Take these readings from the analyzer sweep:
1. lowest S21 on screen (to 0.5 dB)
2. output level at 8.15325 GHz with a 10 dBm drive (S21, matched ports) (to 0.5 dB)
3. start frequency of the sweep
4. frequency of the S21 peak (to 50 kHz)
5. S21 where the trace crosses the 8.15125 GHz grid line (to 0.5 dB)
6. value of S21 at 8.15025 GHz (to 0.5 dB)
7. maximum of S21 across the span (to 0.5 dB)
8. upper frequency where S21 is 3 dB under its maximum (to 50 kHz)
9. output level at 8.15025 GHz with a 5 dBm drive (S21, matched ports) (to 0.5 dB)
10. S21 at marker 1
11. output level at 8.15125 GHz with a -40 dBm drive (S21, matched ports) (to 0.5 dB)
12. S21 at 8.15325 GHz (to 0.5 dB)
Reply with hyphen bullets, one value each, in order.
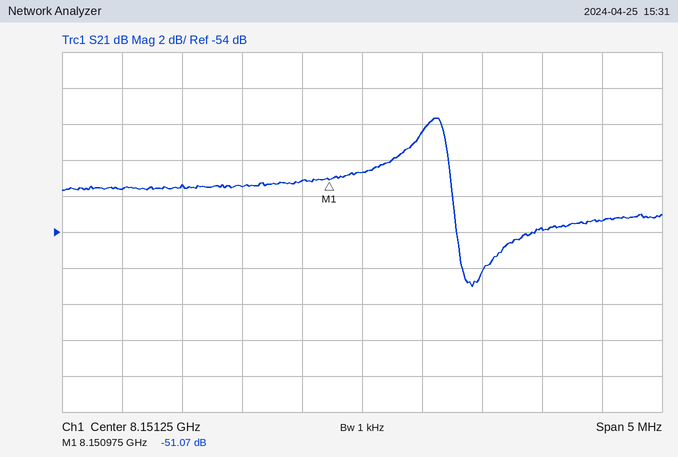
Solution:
- -57.0 dB
- -43.5 dBm
- 8.14875 GHz
- 8.15185 GHz
- -50.5 dB
- -51.5 dB
- -47.5 dB
- 8.15200 GHz
- -46.5 dBm
- -51.07 dB
- -90.5 dBm
- -53.5 dB
